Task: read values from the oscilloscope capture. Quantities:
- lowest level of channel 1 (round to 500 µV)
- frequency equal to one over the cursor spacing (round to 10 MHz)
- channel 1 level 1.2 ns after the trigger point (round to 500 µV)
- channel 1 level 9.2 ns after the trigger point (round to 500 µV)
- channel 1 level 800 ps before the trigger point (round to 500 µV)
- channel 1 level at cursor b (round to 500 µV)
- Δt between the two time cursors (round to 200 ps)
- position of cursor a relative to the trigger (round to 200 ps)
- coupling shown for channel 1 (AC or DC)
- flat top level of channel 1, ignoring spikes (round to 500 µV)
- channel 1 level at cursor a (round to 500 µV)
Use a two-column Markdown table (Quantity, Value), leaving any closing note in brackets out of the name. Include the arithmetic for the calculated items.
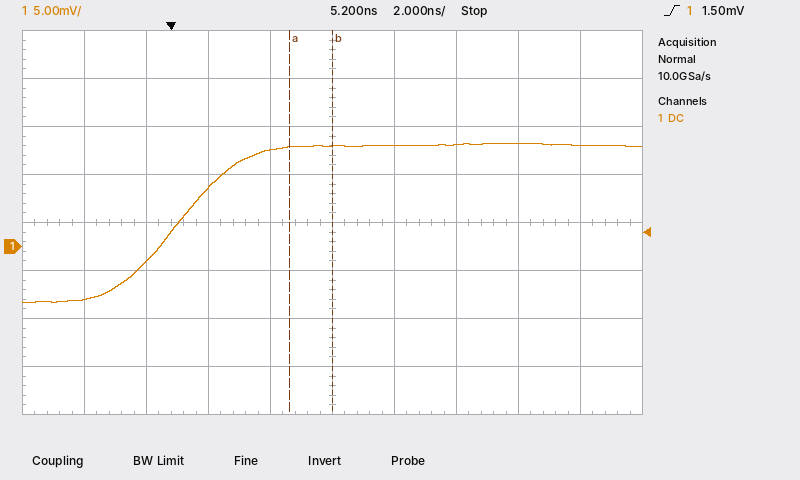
| Quantity | Value |
|---|---|
| lowest level of channel 1 | -6.0 mV |
| frequency equal to one over the cursor spacing | 1 / 1.4 ns ≈ 710 MHz |
| channel 1 level 1.2 ns after the trigger point | 6.0 mV |
| channel 1 level 9.2 ns after the trigger point | 10.5 mV |
| channel 1 level 800 ps before the trigger point | -1.5 mV |
| channel 1 level at cursor b | 10.5 mV |
| Δt between the two time cursors | 1.4 ns |
| position of cursor a relative to the trigger | +3.8 ns |
| coupling shown for channel 1 | DC |
| flat top level of channel 1, ignoring spikes | 10.5 mV |
| channel 1 level at cursor a | 10.5 mV |
